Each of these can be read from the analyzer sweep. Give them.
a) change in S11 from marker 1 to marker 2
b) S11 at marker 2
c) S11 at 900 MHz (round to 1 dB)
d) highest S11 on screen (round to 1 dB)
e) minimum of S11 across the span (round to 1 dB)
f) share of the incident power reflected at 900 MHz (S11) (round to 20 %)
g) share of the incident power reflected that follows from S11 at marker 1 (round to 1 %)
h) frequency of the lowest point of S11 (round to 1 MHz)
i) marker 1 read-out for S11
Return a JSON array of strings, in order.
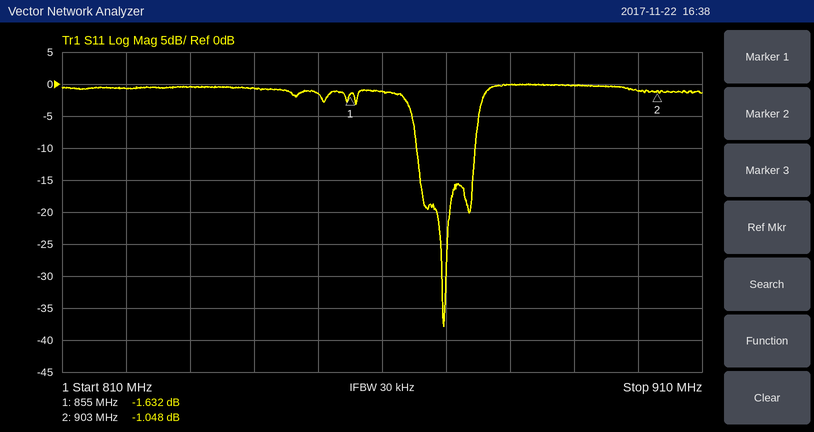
["0.584 dB", "-1.048 dB", "-1 dB", "0 dB", "-38 dB", "80 %", "69 %", "870 MHz", "-1.632 dB"]
